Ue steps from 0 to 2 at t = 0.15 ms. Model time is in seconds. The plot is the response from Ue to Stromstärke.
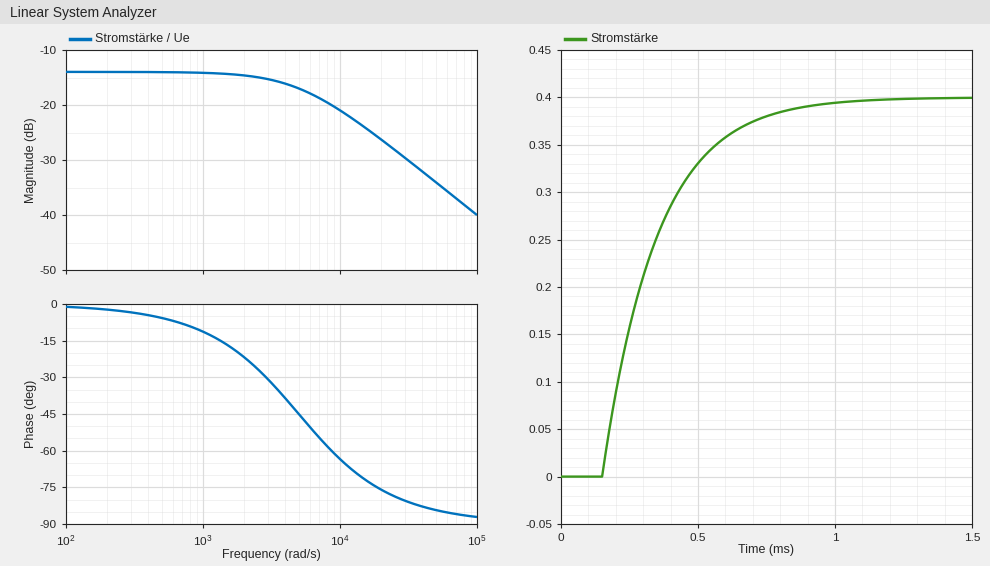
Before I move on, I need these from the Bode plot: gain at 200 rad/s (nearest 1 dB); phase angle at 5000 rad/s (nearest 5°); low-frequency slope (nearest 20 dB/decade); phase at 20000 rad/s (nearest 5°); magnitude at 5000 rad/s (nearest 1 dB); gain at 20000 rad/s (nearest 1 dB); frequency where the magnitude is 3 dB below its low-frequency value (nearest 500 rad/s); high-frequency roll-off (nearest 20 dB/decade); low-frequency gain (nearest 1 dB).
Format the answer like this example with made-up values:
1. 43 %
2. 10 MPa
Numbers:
1. -14 dB
2. -45°
3. 0 dB/decade
4. -75°
5. -17 dB
6. -26 dB
7. 5000 rad/s
8. -20 dB/decade
9. -14 dB
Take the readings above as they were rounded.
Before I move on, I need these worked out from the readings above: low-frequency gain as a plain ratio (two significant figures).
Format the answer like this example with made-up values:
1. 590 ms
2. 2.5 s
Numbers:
1. 0.20
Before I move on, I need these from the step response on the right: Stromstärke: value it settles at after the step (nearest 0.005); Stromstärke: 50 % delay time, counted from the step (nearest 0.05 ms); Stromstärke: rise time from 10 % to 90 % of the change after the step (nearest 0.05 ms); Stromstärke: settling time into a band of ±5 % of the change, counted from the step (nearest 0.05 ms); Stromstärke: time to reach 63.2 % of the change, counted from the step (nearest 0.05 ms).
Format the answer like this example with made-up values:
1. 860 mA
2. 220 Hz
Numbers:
1. 0.400
2. 0.15 ms
3. 0.45 ms
4. 0.60 ms
5. 0.20 ms
